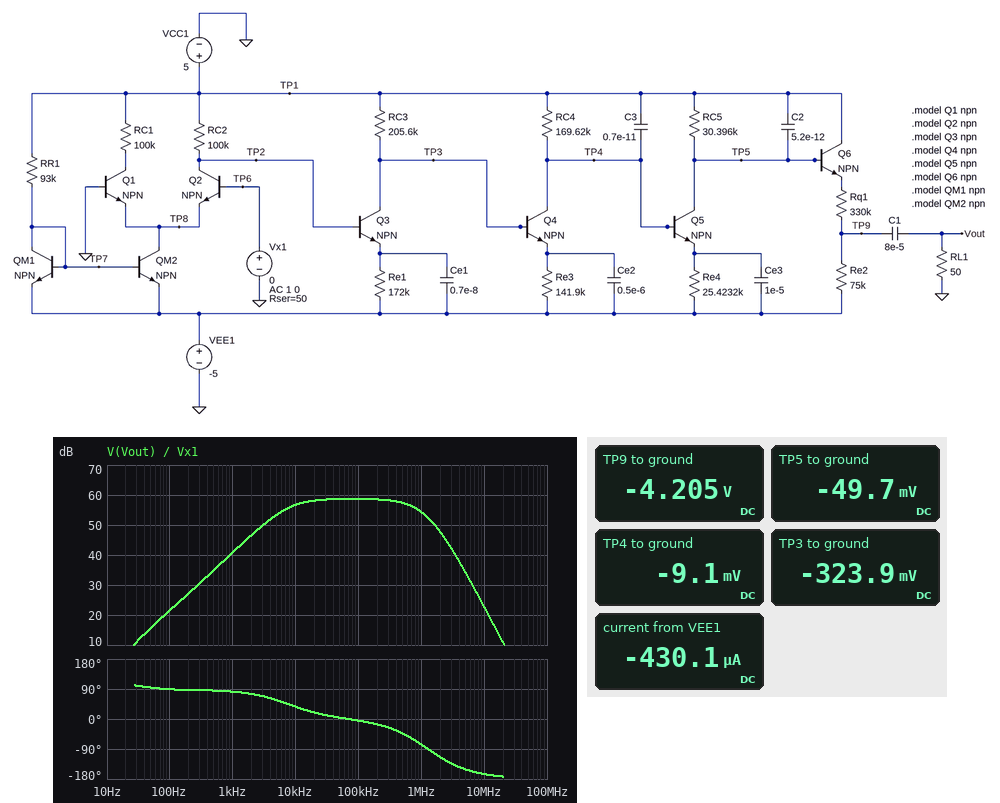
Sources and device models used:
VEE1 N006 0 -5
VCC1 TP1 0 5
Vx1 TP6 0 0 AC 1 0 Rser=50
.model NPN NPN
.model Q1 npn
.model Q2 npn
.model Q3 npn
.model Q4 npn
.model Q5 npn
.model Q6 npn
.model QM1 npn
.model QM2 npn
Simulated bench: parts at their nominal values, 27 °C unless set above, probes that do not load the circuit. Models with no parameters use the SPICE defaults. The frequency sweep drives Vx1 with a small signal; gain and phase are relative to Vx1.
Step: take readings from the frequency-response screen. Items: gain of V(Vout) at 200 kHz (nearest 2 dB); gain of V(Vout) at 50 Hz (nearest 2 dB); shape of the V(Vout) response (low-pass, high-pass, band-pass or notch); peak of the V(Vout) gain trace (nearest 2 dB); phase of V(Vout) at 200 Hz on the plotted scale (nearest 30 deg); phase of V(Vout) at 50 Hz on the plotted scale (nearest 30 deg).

58 dB
16 dB
band-pass
58 dB
90 deg
90 deg
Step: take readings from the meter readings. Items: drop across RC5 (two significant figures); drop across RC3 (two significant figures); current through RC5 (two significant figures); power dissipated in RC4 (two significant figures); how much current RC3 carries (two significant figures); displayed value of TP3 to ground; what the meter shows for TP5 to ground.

5.0 V
5.3 V
170 µA
150 µW
26 µA
-323.9 mV
-49.7 mV
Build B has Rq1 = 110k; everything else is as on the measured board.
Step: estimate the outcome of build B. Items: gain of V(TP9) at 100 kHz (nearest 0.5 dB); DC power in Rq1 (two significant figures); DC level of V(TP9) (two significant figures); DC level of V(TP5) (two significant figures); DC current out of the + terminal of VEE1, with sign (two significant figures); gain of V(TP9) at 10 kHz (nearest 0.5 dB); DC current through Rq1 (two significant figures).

68.0 dB
59 µW
-3.3 V
-53 mV
-440 µA
66.0 dB
23 µA
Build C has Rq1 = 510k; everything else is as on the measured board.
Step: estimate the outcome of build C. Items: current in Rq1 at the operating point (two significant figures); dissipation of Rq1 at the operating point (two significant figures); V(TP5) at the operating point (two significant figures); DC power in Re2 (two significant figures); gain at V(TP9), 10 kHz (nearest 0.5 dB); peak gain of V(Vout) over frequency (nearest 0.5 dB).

7.4 µA
28 µW
-49 mV
4.1 µW
53.0 dB
55.0 dB
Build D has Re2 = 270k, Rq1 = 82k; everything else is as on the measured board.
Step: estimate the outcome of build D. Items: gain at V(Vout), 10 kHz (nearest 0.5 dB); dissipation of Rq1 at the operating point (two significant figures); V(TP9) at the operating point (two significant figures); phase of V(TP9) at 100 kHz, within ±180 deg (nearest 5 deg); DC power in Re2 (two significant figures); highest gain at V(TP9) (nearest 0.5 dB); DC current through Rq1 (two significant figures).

68.5 dB
12 µW
-1.7 V
-5 deg
40 µW
70.5 dB
12 µA
